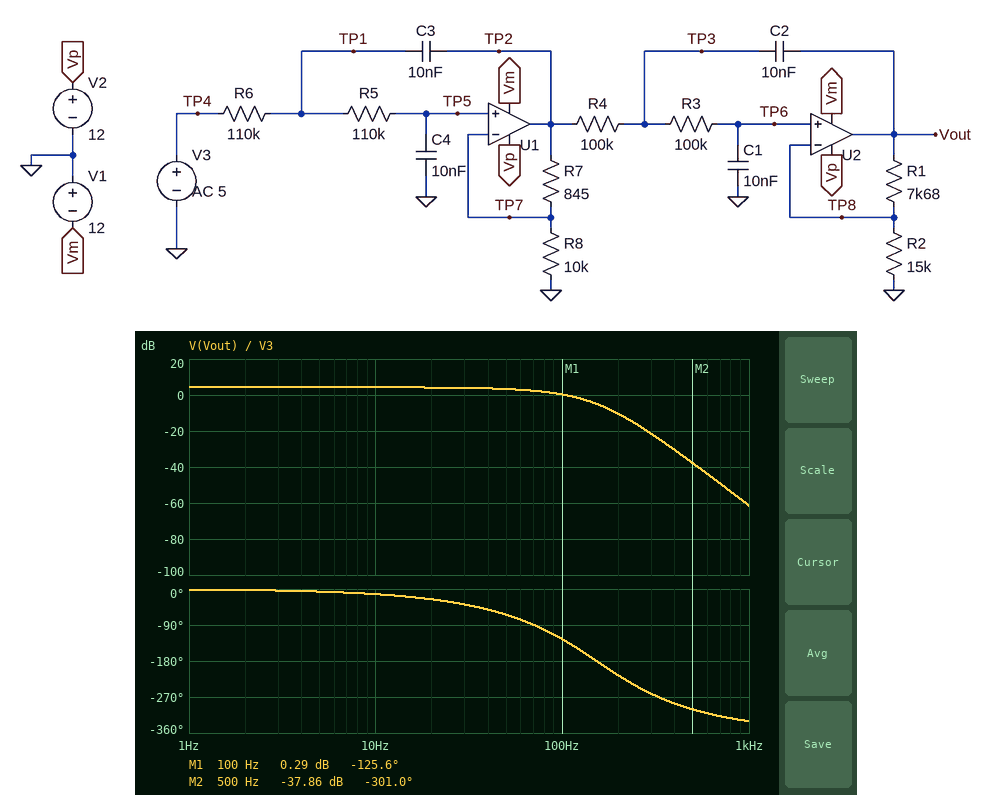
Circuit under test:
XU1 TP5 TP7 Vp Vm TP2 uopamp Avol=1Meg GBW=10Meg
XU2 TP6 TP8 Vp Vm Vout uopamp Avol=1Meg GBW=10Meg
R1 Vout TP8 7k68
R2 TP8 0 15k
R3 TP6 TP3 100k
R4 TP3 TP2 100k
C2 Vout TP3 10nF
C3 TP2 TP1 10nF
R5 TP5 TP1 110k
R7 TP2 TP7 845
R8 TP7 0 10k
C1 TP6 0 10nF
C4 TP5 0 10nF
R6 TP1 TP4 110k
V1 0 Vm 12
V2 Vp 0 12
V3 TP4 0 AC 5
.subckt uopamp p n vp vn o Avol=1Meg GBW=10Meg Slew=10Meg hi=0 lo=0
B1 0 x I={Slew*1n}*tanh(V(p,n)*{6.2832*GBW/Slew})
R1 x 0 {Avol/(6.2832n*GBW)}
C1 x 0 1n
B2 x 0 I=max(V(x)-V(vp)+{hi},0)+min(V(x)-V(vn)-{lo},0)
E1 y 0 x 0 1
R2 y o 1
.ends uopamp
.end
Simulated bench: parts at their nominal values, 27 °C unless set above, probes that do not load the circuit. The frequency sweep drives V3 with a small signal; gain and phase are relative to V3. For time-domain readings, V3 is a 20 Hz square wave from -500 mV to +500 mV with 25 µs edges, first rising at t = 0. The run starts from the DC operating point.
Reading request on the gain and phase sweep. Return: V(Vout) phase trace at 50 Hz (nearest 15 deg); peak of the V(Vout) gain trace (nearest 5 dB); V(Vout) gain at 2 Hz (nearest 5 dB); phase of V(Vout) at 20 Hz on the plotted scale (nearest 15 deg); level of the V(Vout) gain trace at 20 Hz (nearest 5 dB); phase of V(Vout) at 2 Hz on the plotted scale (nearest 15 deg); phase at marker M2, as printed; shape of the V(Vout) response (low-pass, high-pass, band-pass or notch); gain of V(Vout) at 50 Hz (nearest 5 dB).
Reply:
-60 deg
5 dB
5 dB
-30 deg
5 dB
0 deg
-301.0 deg
low-pass
5 dB
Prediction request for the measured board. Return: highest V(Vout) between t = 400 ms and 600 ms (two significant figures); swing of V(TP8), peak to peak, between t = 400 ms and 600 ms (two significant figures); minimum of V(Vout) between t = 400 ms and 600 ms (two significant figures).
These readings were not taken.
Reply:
820 mV
1.1 V
-820 mV
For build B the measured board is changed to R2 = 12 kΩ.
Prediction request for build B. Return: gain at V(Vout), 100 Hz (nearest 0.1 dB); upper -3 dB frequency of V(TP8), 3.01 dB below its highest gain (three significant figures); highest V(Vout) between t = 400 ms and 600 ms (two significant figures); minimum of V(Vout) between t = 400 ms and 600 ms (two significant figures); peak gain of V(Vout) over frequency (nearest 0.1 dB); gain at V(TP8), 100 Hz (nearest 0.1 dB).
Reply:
1.5 dB
93.6 Hz
900 mV
-900 mV
5.0 dB
-2.8 dB
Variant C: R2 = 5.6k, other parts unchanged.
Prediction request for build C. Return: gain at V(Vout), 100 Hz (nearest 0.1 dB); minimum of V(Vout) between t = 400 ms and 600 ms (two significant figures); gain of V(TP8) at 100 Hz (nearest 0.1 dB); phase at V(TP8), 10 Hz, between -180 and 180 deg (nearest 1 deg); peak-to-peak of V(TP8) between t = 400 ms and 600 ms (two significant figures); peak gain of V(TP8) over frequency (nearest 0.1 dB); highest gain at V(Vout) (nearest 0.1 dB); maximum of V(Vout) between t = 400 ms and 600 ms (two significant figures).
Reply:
8.0 dB
-1.6 V
0.5 dB
-10 deg
1.3 V
0.7 dB
8.2 dB
1.6 V
